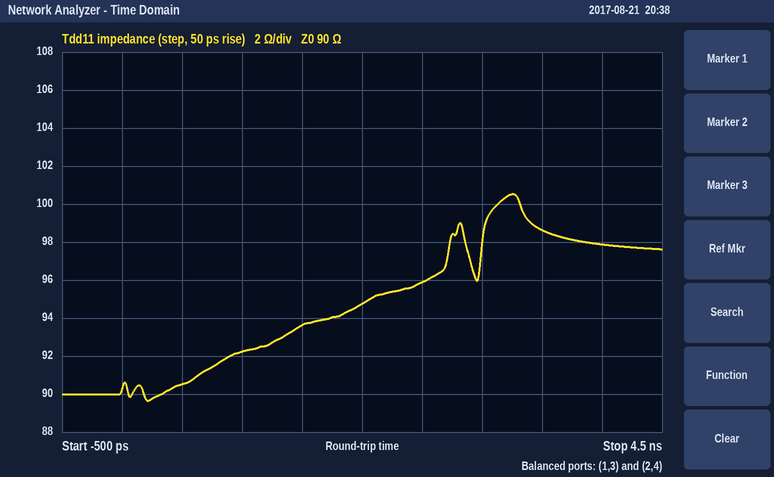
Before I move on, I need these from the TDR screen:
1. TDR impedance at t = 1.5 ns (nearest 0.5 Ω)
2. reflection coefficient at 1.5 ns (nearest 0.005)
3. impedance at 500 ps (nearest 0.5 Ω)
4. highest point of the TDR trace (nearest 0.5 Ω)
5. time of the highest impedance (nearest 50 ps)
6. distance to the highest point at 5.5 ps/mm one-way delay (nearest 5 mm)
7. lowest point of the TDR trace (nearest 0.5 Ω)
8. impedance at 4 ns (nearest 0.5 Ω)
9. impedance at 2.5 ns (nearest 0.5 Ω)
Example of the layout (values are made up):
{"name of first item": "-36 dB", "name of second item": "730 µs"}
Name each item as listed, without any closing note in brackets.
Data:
{"TDR impedance at t = 1.5 ns": "93.5 Ω", "reflection coefficient at 1.5 ns": "+0.020", "impedance at 500 ps": "90.5 Ω", "highest point of the TDR trace": "100.5 Ω", "time of the highest impedance": "3.25 ns", "distance to the highest point at 5.5 ps/mm one-way delay": "295 mm", "lowest point of the TDR trace": "89.5 Ω", "impedance at 4 ns": "98.0 Ω", "impedance at 2.5 ns": "96.0 Ω"}
